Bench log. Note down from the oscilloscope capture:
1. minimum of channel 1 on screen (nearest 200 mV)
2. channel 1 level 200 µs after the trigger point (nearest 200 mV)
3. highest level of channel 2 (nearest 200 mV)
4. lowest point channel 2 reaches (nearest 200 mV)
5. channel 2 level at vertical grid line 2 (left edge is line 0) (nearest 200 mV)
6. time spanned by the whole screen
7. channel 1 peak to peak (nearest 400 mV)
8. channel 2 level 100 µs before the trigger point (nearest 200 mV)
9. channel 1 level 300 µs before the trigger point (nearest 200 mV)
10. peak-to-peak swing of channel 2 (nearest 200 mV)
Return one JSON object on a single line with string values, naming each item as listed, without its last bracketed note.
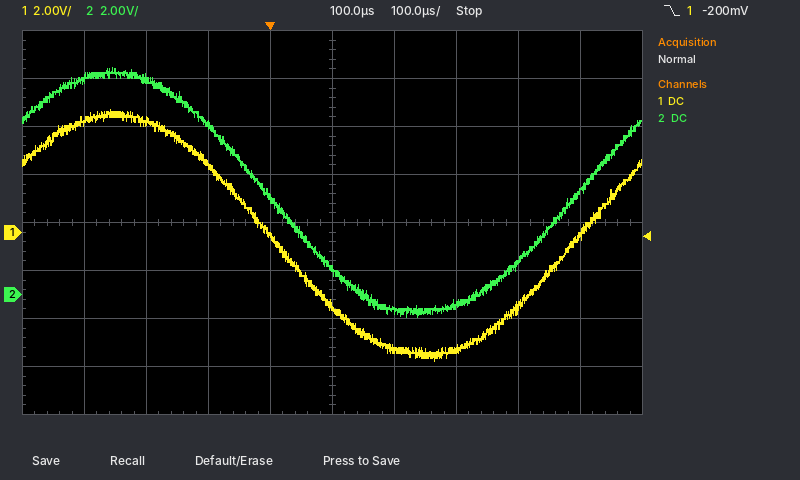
{"minimum of channel 1 on screen": "-5.4 V", "channel 1 level 200 µs after the trigger point": "-4.8 V", "highest level of channel 2": "9.4 V", "lowest point channel 2 reaches": "-1.0 V", "channel 2 level at vertical grid line 2 (left edge is line 0)": "9.0 V", "time spanned by the whole screen": "1 ms", "channel 1 peak to peak": "10.4 V", "channel 2 level 100 µs before the trigger point": "7.0 V", "channel 1 level 300 µs before the trigger point": "4.6 V", "peak-to-peak swing of channel 2": "10.4 V"}
